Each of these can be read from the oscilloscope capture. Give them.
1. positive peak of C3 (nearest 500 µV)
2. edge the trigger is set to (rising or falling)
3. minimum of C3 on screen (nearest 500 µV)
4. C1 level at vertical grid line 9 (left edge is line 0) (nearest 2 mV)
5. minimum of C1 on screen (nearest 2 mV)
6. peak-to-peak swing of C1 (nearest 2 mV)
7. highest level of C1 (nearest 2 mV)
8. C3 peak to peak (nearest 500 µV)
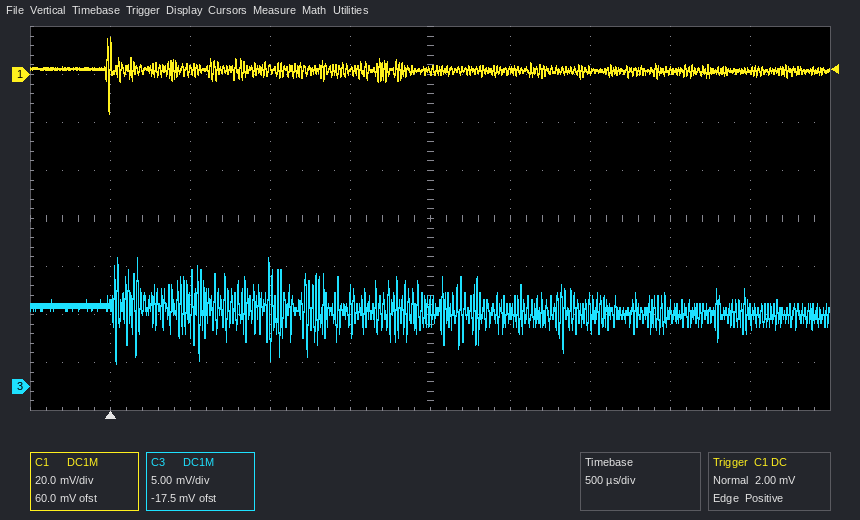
13.5 mV
rising
2.5 mV
2 mV
-16 mV
32 mV
16 mV
11.0 mV
